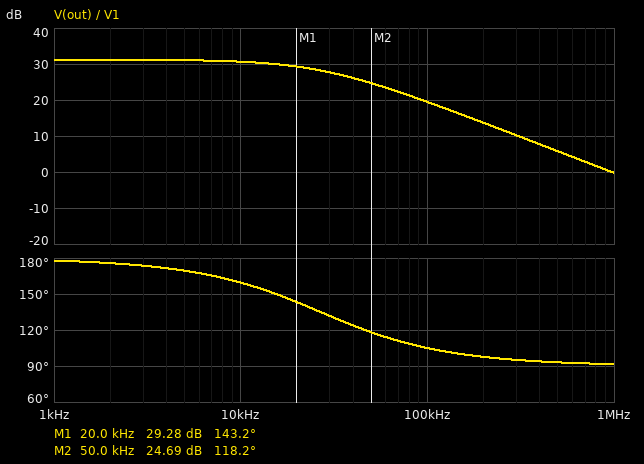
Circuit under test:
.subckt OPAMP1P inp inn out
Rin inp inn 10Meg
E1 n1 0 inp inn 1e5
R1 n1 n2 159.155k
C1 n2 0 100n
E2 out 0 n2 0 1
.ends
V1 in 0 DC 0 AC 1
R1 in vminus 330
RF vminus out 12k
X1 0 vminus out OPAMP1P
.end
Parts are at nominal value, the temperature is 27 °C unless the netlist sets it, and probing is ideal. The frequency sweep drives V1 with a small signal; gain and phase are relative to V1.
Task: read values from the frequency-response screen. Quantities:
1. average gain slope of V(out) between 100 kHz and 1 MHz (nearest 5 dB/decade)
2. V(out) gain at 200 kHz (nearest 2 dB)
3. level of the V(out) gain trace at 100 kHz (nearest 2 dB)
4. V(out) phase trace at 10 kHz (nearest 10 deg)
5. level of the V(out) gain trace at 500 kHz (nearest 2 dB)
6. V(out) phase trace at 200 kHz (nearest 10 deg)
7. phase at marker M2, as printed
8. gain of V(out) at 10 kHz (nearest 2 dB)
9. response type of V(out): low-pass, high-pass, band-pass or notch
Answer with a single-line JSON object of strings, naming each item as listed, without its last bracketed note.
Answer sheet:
{"average gain slope of V(out) between 100 kHz and 1 MHz": "-20 dB/decade", "V(out) gain at 200 kHz": "14 dB", "level of the V(out) gain trace at 100 kHz": "20 dB", "V(out) phase trace at 10 kHz": "160 deg", "level of the V(out) gain trace at 500 kHz": "6 dB", "V(out) phase trace at 200 kHz": "100 deg", "phase at marker M2, as printed": "118.2 deg", "gain of V(out) at 10 kHz": "30 dB", "response type of V(out): low-pass, high-pass, band-pass or notch": "low-pass"}
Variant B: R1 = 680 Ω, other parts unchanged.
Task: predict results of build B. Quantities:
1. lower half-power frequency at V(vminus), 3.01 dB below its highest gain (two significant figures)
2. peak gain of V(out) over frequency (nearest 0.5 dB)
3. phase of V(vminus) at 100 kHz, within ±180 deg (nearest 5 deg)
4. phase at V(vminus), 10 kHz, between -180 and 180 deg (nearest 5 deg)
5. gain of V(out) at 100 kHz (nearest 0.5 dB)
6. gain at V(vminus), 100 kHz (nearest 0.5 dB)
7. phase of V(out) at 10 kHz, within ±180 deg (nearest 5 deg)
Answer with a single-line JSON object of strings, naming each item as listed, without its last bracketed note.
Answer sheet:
{"lower half-power frequency at V(vminus), 3.01 dB below its highest gain": "54 kHz", "peak gain of V(out) over frequency": "25.0 dB", "phase of V(vminus) at 100 kHz, within ±180 deg": "30 deg", "phase at V(vminus), 10 kHz, between -180 and 180 deg": "80 deg", "gain of V(out) at 100 kHz": "18.5 dB", "gain at V(vminus), 100 kHz": "-1.5 dB", "phase of V(out) at 10 kHz, within ±180 deg": "170 deg"}
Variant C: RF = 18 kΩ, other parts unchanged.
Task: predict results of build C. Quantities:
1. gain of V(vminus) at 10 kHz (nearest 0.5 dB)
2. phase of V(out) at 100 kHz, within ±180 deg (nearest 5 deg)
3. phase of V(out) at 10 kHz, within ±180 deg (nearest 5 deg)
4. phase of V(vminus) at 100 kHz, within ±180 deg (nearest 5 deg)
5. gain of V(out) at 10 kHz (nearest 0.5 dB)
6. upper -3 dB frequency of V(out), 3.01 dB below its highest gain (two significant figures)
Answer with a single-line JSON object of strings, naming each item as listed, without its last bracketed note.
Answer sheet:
{"gain of V(vminus) at 10 kHz": "-6.5 dB", "phase of V(out) at 100 kHz, within ±180 deg": "100 deg", "phase of V(out) at 10 kHz, within ±180 deg": "150 deg", "phase of V(vminus) at 100 kHz, within ±180 deg": "10 deg", "gain of V(out) at 10 kHz": "33.5 dB", "upper -3 dB frequency of V(out), 3.01 dB below its highest gain": "18 kHz"}
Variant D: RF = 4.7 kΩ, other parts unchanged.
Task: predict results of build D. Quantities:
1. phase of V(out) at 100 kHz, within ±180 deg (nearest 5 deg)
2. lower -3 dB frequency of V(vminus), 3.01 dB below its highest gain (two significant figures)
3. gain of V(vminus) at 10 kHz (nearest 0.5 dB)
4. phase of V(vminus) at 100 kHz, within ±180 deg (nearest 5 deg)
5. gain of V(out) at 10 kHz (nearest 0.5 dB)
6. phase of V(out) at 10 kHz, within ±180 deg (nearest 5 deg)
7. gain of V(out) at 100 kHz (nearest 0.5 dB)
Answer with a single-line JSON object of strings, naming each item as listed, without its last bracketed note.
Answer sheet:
{"phase of V(out) at 100 kHz, within ±180 deg": "125 deg", "lower -3 dB frequency of V(vminus), 3.01 dB below its highest gain": "66 kHz", "gain of V(vminus) at 10 kHz": "-17.0 dB", "phase of V(vminus) at 100 kHz, within ±180 deg": "35 deg", "gain of V(out) at 10 kHz": "23.0 dB", "phase of V(out) at 10 kHz, within ±180 deg": "170 deg", "gain of V(out) at 100 kHz": "18.0 dB"}
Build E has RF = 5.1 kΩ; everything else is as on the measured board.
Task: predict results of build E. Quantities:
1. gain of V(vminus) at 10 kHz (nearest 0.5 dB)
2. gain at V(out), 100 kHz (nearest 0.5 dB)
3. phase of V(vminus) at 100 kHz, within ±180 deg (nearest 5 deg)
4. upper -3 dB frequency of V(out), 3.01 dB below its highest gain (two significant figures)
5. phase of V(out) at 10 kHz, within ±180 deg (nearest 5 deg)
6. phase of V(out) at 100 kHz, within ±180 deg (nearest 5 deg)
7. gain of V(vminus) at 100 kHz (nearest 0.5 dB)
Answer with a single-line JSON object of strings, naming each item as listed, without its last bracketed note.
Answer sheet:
{"gain of V(vminus) at 10 kHz": "-16.5 dB", "gain at V(out), 100 kHz": "18.0 dB", "phase of V(vminus) at 100 kHz, within ±180 deg": "30 deg", "upper -3 dB frequency of V(out), 3.01 dB below its highest gain": "61 kHz", "phase of V(out) at 10 kHz, within ±180 deg": "170 deg", "phase of V(out) at 100 kHz, within ±180 deg": "120 deg", "gain of V(vminus) at 100 kHz": "-2.0 dB"}
